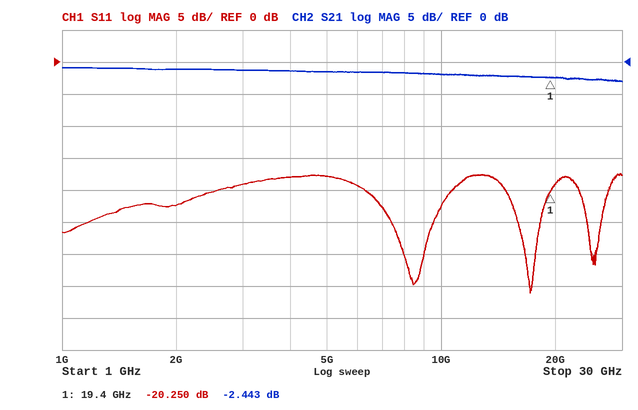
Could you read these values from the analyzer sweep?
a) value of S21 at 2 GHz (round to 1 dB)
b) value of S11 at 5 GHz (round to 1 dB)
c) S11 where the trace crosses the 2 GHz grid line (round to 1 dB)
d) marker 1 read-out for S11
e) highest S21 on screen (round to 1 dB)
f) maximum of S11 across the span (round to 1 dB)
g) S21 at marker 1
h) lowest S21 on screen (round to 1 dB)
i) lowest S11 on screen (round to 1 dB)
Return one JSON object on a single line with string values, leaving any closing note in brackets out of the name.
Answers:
{"value of S21 at 2 GHz": "-1 dB", "value of S11 at 5 GHz": "-18 dB", "S11 where the trace crosses the 2 GHz grid line": "-22 dB", "marker 1 read-out for S11": "-20.250 dB", "highest S21 on screen": "-1 dB", "maximum of S11 across the span": "-17 dB", "S21 at marker 1": "-2.443 dB", "lowest S21 on screen": "-3 dB", "lowest S11 on screen": "-36 dB"}
